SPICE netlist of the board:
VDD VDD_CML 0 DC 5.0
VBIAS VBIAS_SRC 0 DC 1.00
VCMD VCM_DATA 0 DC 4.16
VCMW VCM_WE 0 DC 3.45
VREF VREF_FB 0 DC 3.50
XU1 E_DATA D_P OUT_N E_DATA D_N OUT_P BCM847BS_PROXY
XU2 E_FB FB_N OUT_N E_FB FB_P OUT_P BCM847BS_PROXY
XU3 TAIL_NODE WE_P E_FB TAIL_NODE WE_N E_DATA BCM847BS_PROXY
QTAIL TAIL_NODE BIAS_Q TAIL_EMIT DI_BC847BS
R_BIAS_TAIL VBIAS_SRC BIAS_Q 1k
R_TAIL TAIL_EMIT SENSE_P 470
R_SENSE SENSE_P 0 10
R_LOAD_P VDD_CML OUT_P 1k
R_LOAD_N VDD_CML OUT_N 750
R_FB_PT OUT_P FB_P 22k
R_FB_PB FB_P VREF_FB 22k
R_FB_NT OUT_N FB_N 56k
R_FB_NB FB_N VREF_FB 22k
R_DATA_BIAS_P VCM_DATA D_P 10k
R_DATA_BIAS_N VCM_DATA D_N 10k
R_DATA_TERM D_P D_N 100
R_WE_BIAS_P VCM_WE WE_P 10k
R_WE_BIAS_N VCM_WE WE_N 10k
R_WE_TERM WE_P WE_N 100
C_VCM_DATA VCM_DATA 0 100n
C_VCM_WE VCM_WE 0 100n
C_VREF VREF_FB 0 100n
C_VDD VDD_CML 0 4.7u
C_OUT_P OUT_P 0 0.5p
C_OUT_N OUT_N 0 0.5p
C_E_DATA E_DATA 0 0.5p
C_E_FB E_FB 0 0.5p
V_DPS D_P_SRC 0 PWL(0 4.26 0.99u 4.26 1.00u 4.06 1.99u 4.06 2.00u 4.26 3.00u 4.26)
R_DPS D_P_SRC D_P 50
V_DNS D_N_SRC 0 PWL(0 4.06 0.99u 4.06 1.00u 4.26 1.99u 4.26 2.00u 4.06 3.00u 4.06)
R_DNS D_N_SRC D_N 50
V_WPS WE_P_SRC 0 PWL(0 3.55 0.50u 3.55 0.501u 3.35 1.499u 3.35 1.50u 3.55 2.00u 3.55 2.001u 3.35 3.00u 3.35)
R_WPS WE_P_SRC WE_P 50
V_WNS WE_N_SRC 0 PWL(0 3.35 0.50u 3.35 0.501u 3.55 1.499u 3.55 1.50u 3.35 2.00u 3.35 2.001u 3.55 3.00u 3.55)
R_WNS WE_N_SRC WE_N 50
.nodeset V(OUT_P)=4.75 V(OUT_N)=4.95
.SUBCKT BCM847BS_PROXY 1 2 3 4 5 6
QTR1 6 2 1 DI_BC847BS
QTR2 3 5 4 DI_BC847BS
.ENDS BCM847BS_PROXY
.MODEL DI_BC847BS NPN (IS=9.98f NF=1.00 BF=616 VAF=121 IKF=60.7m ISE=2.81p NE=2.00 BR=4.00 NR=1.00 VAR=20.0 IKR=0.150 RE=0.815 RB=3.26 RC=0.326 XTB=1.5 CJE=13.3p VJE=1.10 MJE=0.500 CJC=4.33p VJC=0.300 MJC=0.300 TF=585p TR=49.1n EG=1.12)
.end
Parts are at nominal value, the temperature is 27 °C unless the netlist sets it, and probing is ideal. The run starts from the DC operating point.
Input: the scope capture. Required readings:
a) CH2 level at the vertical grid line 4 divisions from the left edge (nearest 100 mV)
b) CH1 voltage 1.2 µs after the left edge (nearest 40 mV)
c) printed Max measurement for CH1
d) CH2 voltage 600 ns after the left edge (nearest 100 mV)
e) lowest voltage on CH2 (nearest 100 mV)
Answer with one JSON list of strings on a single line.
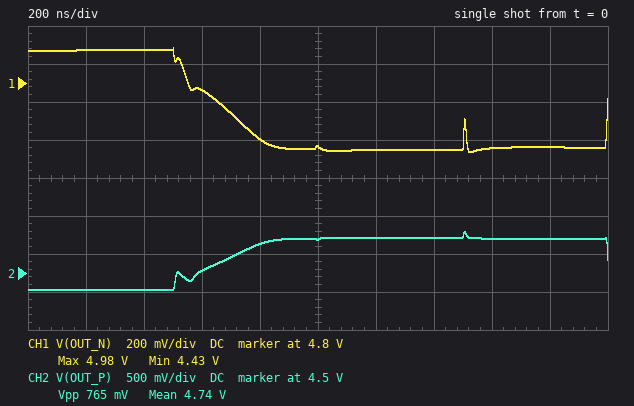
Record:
["4.9 V", "4.44 V", "4.98 V", "4.5 V", "4.3 V"]
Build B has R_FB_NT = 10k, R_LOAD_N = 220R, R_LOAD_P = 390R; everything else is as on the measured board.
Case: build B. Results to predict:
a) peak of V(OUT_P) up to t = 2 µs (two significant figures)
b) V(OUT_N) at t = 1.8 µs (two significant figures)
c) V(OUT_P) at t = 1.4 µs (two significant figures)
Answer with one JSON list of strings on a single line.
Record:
["5.0 V", "4.8 V", "4.7 V"]
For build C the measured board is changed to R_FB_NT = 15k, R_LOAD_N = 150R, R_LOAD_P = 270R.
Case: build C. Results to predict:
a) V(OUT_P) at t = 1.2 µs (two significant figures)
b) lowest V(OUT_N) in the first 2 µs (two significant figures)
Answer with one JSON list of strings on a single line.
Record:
["4.8 V", "4.9 V"]
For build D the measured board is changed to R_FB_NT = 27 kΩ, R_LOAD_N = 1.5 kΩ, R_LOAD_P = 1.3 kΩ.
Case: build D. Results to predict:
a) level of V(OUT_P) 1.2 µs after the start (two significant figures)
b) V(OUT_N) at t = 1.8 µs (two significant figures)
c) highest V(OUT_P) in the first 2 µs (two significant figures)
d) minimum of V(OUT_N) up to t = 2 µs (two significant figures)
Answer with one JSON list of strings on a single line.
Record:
["4.1 V", "4.0 V", "4.9 V", "3.9 V"]
